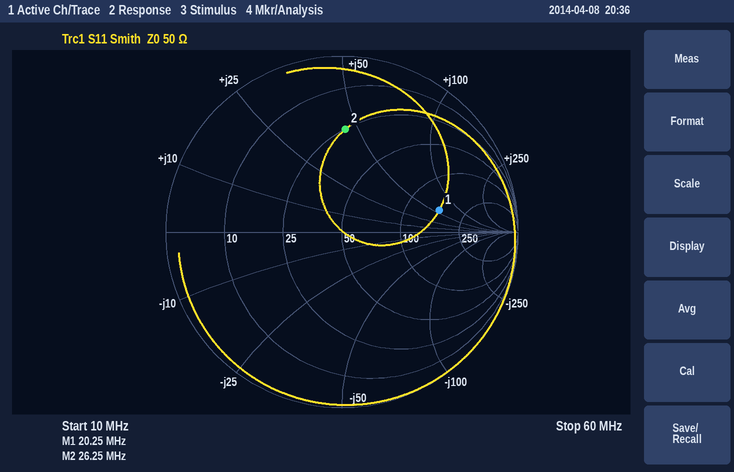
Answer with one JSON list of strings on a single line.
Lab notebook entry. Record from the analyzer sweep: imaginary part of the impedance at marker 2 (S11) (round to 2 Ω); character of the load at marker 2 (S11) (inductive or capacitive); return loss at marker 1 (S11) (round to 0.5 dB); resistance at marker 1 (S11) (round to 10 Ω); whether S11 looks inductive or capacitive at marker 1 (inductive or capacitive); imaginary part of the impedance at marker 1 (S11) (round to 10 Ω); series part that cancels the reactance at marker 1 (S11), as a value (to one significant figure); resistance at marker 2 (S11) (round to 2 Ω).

["+44 Ω", "inductive", "5.0 dB", "160 Ω", "inductive", "+60 Ω", "100 pF", "26 Ω"]
